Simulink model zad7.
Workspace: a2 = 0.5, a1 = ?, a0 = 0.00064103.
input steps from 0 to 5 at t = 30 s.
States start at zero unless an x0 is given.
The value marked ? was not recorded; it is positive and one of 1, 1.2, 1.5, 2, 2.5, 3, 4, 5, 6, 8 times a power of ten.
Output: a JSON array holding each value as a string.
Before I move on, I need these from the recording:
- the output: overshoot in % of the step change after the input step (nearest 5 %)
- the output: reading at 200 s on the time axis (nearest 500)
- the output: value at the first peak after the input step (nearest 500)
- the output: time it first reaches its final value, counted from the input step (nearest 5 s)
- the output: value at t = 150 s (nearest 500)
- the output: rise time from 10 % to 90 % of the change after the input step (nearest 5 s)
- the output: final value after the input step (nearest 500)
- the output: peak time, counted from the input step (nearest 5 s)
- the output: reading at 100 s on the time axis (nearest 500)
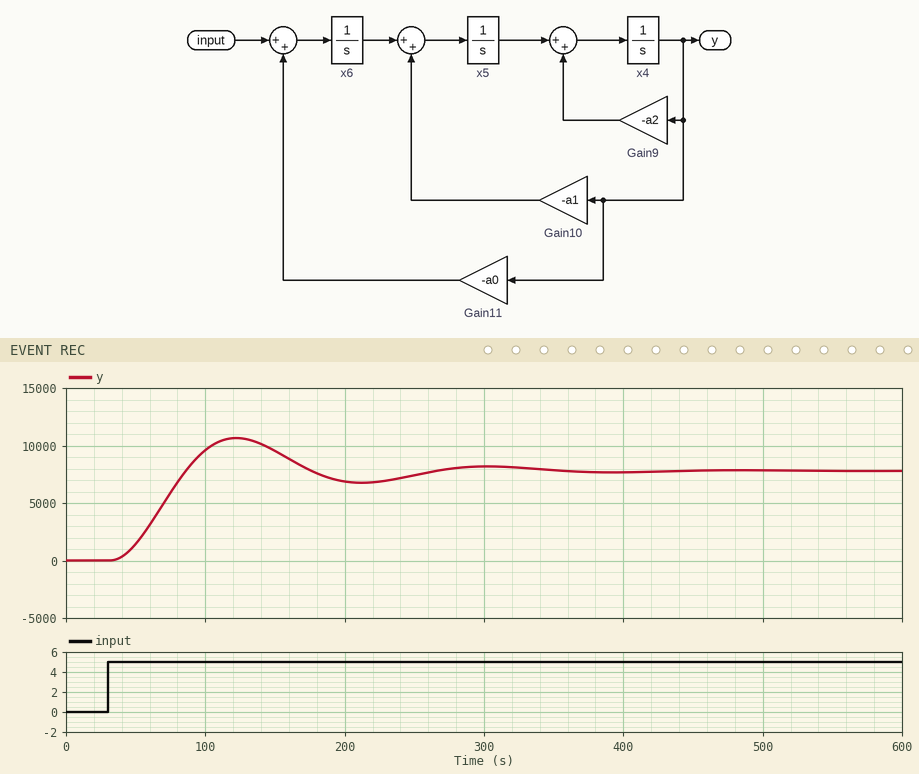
["35 %", "7000", "10500", "55 s", "9500", "35 s", "8000", "90 s", "9500"]
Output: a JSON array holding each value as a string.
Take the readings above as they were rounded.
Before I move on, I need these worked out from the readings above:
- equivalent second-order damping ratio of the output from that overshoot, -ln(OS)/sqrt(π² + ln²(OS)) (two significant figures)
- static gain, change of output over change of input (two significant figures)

["0.32", "1600"]
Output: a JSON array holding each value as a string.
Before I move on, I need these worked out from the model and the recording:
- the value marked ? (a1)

["0.012"]
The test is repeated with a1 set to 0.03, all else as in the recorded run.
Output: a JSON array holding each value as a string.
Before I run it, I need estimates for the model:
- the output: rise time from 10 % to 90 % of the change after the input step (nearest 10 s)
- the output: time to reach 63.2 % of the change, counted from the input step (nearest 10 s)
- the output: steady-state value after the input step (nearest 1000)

["70 s", "50 s", "8000"]
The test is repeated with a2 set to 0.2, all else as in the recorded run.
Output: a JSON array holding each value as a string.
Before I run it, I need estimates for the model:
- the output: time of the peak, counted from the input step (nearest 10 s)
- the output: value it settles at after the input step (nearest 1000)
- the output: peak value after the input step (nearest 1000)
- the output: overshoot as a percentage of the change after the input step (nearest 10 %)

["60 s", "8000", "10000", "20 %"]
